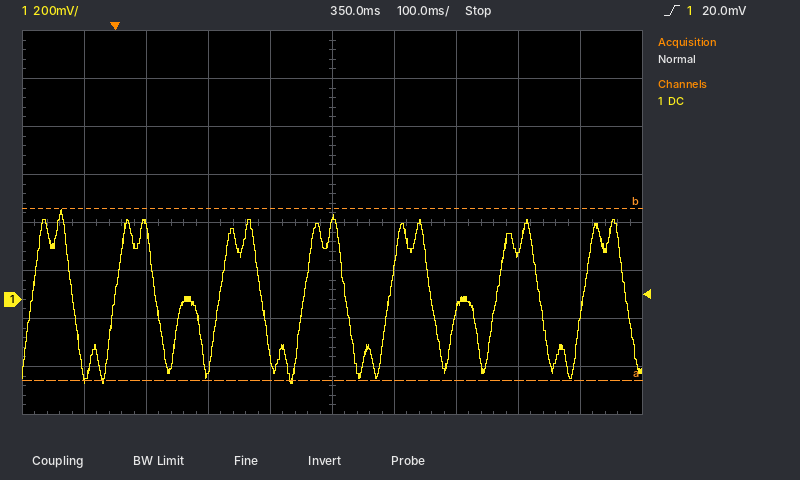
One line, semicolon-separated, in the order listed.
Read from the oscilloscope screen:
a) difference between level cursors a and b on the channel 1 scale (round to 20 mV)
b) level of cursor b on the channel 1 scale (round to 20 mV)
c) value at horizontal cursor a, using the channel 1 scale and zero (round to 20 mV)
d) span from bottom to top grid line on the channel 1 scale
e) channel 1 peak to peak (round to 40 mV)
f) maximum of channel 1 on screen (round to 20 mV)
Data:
720 mV; 380 mV; -340 mV; 1.6 V; 720 mV; 380 mV
